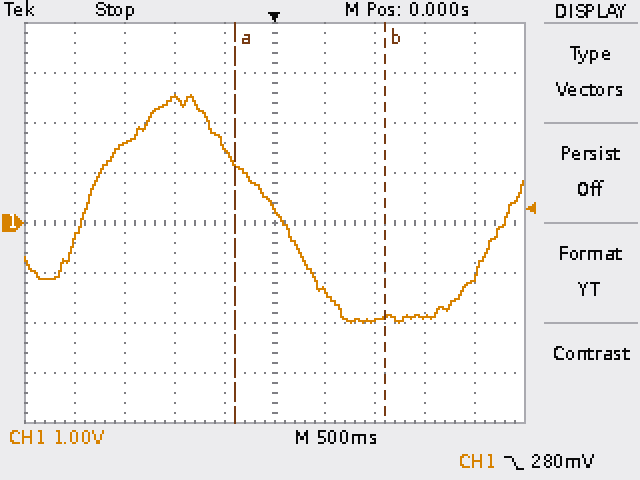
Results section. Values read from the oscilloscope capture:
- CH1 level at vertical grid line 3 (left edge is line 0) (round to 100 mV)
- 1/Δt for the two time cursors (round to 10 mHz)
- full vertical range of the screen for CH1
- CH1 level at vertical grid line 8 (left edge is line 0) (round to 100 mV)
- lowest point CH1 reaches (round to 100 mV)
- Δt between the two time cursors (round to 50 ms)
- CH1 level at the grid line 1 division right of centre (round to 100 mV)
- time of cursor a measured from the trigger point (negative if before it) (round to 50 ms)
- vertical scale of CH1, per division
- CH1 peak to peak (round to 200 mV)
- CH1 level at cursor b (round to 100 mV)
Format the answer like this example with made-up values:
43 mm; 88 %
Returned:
2.5 V; 670 mHz; 8 V; -1.9 V; -2.0 V; 1.50 s; -1.4 V; -400 ms; 1 V; 4.6 V; -1.9 V
